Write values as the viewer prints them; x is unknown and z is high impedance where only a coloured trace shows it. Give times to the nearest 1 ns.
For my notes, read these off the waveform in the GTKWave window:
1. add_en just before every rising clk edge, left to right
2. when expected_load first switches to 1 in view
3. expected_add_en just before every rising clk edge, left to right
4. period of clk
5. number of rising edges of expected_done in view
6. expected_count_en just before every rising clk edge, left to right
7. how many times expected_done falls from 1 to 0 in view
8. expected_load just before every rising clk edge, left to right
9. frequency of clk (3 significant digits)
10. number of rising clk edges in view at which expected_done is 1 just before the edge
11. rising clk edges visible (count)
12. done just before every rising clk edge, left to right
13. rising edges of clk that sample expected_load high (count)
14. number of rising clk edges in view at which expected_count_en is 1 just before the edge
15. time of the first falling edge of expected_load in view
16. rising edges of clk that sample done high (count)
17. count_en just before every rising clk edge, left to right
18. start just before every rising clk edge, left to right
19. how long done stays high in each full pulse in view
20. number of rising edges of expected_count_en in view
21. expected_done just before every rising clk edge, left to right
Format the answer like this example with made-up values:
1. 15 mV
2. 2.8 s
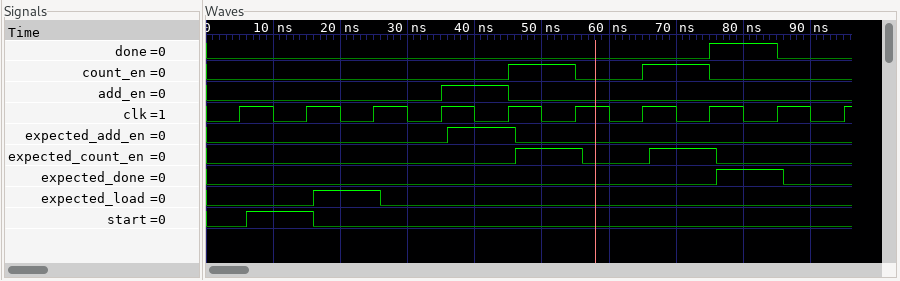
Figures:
1. 0 0 0 0 1 0 0 0 0 0
2. 16 ns
3. 0 0 0 0 1 0 0 0 0 0
4. 10 ns
5. 1
6. 0 0 0 0 0 1 0 1 0 0
7. 1
8. 0 0 1 0 0 0 0 0 0 0
9. 100 MHz
10. 1
11. 10
12. 0 0 0 0 0 0 0 0 1 0
13. 1
14. 2
15. 26 ns
16. 1
17. 0 0 0 0 0 1 0 1 0 0
18. 0 1 0 0 0 0 0 0 0 0
19. 10 ns
20. 2
21. 0 0 0 0 0 0 0 0 1 0
